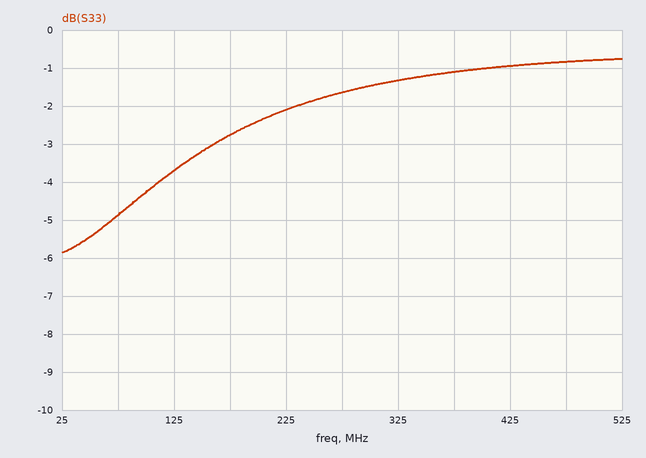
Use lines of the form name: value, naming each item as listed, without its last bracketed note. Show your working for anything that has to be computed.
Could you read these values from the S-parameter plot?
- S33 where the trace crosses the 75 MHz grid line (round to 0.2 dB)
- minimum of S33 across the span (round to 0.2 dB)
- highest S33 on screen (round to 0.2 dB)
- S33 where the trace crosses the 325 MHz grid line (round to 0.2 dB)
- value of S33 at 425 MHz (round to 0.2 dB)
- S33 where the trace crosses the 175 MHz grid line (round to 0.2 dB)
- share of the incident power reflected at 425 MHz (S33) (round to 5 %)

S33 where the trace crosses the 75 MHz grid line: -4.8 dB
minimum of S33 across the span: -5.8 dB
highest S33 on screen: -0.8 dB
S33 where the trace crosses the 325 MHz grid line: -1.4 dB
value of S33 at 425 MHz: -1.0 dB
S33 where the trace crosses the 175 MHz grid line: -2.8 dB
share of the incident power reflected at 425 MHz (S33): 10^(-1/10) ≈ 79.4 %, so 80 % to the nearest 5 %
